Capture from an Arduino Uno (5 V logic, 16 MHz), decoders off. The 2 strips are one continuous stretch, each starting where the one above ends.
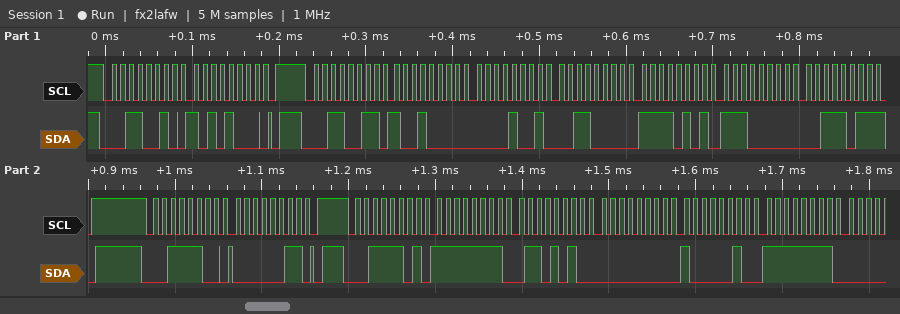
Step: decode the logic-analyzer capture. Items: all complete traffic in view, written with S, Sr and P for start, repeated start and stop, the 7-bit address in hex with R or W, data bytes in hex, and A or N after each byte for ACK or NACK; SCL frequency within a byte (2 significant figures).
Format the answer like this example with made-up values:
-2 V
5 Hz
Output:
S 19W A A8 A P S 19R A 90 A 09 A 30 A F5 A E0 A 3B N P S 1EW A 03 A P S 1ER A FF A 6A A 00 A 82 A FF A
100 kHz
